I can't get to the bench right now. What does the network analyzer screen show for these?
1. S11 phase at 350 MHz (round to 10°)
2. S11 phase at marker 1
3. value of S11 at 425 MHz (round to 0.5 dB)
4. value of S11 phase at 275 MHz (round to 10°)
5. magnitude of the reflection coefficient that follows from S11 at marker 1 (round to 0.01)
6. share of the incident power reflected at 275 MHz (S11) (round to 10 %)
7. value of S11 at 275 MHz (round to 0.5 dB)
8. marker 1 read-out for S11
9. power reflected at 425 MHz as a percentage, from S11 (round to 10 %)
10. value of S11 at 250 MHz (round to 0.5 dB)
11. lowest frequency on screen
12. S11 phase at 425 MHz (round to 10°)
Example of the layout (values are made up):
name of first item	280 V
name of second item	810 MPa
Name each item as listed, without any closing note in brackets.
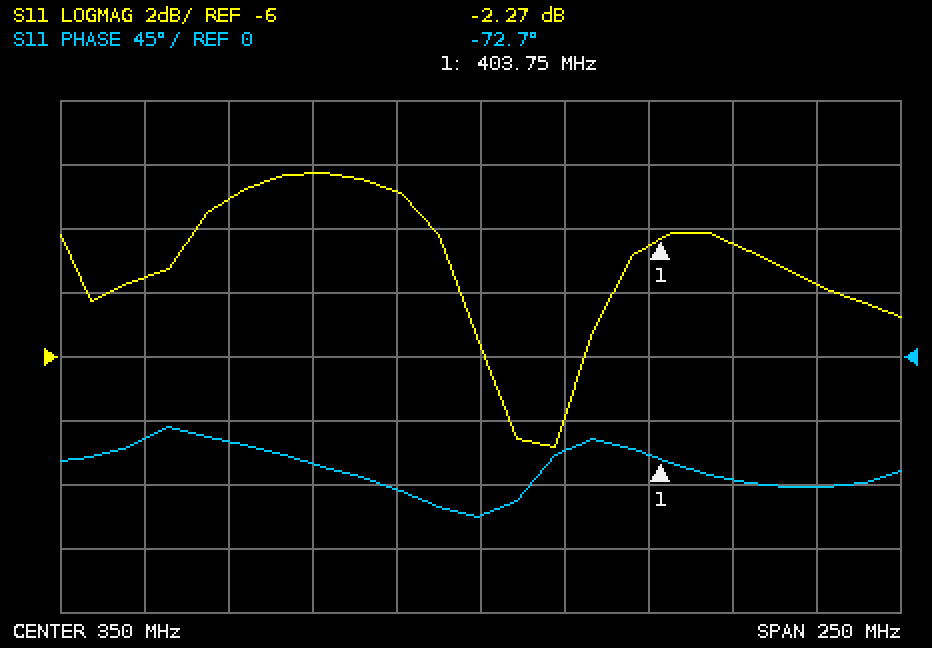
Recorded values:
S11 phase at 350 MHz	-110°
S11 phase at marker 1	-72.7°
value of S11 at 425 MHz	-2.5 dB
value of S11 phase at 275 MHz	-60°
magnitude of the reflection coefficient that follows from S11 at marker 1	0.77
share of the incident power reflected at 275 MHz (S11)	80 %
value of S11 at 275 MHz	-1.0 dB
marker 1 read-out for S11	-2.27 dB
power reflected at 425 MHz as a percentage, from S11	60 %
value of S11 at 250 MHz	-3.5 dB
lowest frequency on screen	225 MHz
S11 phase at 425 MHz	-90°
